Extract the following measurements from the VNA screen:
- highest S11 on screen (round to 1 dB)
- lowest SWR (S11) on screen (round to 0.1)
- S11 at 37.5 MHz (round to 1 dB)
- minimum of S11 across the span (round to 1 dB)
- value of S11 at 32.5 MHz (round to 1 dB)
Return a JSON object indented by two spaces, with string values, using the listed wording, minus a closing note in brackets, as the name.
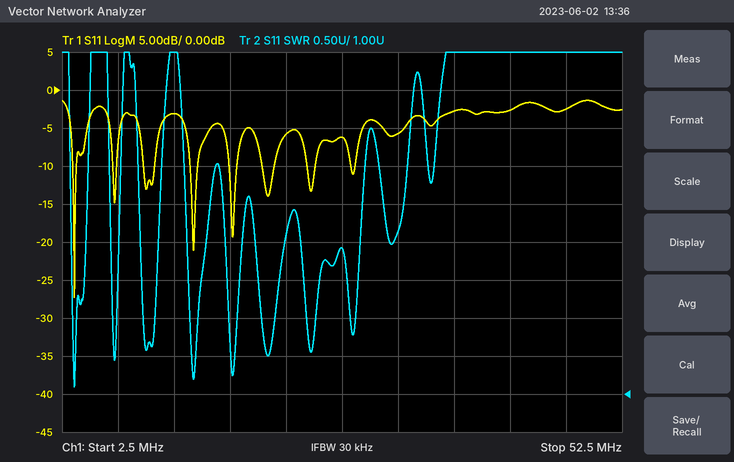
{
  "highest S11 on screen": "-1 dB",
  "lowest SWR (S11) on screen": "1.1",
  "S11 at 37.5 MHz": "-3 dB",
  "minimum of S11 across the span": "-27 dB",
  "value of S11 at 32.5 MHz": "-6 dB"
}
